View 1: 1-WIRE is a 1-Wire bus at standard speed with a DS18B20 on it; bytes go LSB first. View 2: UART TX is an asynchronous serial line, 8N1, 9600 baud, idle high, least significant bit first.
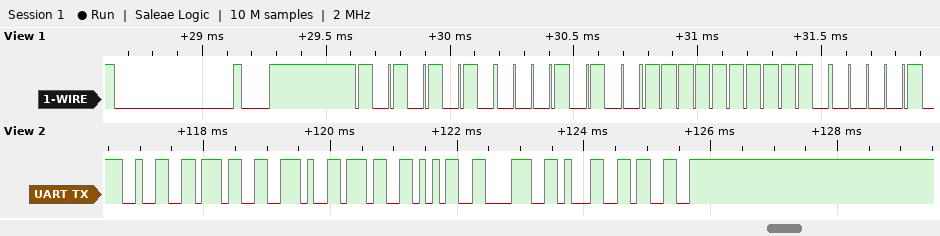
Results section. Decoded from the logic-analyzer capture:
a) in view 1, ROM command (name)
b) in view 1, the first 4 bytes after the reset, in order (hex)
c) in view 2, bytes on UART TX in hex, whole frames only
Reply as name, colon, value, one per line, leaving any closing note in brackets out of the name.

in view 1, ROM command: Match ROM
in view 1, the first 4 bytes after the reset, in order: 55 28 FF 83
in view 2, bytes on UART TX in hex, whole frames only: 32 37 2E 37 35 38 31 33
